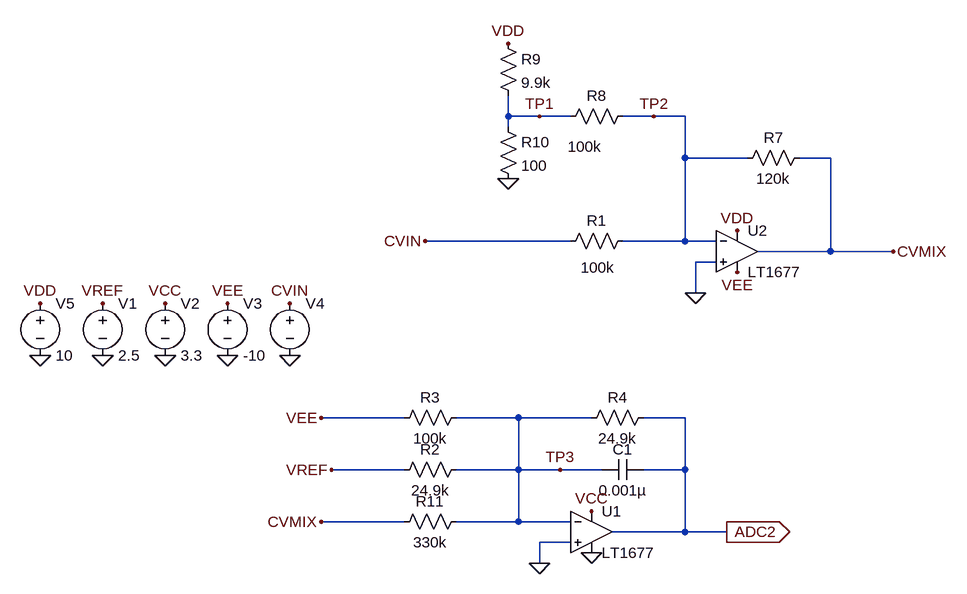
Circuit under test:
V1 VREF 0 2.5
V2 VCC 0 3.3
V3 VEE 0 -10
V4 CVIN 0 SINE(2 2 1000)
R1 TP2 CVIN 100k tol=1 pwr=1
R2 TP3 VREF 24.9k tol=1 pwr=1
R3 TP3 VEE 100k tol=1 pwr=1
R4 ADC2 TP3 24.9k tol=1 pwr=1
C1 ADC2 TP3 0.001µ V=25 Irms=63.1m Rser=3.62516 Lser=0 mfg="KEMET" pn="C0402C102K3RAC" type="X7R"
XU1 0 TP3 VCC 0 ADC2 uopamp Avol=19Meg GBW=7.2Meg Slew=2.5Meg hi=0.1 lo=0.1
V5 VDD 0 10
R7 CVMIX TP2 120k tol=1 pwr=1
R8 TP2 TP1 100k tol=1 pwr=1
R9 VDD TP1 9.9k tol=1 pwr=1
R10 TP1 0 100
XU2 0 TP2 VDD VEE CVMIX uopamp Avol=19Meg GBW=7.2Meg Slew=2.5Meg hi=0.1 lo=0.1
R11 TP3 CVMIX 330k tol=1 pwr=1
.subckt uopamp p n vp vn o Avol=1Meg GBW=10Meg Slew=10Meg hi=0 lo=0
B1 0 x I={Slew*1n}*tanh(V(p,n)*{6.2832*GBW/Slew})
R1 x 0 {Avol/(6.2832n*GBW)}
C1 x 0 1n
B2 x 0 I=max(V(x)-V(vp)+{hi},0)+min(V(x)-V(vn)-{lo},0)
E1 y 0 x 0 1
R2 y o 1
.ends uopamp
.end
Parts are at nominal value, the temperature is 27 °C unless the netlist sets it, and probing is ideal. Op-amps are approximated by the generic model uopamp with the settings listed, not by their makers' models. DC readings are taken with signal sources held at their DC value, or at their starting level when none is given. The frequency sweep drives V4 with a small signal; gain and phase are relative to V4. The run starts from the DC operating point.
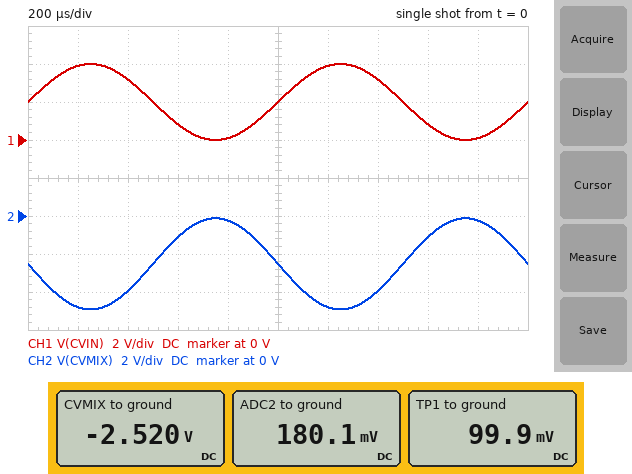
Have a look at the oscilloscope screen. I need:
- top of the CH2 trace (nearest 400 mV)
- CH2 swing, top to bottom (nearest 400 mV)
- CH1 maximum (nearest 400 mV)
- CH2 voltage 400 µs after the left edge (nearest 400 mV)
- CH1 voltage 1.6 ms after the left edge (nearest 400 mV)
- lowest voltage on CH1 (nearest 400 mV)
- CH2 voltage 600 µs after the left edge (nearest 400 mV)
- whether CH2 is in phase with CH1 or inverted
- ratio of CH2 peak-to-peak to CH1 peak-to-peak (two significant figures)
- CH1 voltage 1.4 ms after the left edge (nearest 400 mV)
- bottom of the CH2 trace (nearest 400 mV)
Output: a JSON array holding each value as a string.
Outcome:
["0 V", "4.8 V", "4.0 V", "-4.0 V", "800 mV", "0 V", "-1.2 V", "inverted", "1.2", "3.2 V", "-4.8 V"]
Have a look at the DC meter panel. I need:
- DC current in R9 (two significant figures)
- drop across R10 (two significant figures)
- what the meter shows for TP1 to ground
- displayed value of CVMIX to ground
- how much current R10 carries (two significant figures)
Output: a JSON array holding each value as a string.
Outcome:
["1.0 mA", "100 mV", "99.9 mV", "-2.520 V", "1.0 mA"]
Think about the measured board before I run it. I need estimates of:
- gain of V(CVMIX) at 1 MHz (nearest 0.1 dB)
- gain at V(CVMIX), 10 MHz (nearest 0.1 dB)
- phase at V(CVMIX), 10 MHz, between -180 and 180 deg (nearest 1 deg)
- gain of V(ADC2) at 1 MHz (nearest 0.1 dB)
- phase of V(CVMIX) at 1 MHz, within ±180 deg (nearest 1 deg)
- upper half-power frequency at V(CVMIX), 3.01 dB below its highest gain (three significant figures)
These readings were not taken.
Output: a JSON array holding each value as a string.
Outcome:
["0.7 dB", "-12.1 dB", "102 deg", "-65.7 dB", "155 deg", "2.12 MHz"]
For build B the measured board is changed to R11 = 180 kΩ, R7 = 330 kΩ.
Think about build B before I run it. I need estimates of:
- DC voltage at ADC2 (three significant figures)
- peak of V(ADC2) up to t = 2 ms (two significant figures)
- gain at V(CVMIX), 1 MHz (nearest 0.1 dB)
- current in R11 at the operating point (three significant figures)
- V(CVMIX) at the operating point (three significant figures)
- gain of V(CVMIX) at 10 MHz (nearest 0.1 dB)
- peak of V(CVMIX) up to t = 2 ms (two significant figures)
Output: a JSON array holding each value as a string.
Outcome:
["949 mV", "1.4 V", "7.1 dB", "38.5 µA", "-6.93 V", "-10.1 dB", "-330 mV"]
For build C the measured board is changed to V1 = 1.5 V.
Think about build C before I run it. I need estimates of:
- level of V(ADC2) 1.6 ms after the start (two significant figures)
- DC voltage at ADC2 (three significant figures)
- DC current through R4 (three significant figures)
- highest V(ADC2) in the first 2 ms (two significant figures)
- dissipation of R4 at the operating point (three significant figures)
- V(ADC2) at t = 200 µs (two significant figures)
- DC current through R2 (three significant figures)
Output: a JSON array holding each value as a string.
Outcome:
["1.1 V", "1.18 V", "47.4 µA", "1.4 V", "55.9 µW", "1.3 V", "60.2 µA"]
